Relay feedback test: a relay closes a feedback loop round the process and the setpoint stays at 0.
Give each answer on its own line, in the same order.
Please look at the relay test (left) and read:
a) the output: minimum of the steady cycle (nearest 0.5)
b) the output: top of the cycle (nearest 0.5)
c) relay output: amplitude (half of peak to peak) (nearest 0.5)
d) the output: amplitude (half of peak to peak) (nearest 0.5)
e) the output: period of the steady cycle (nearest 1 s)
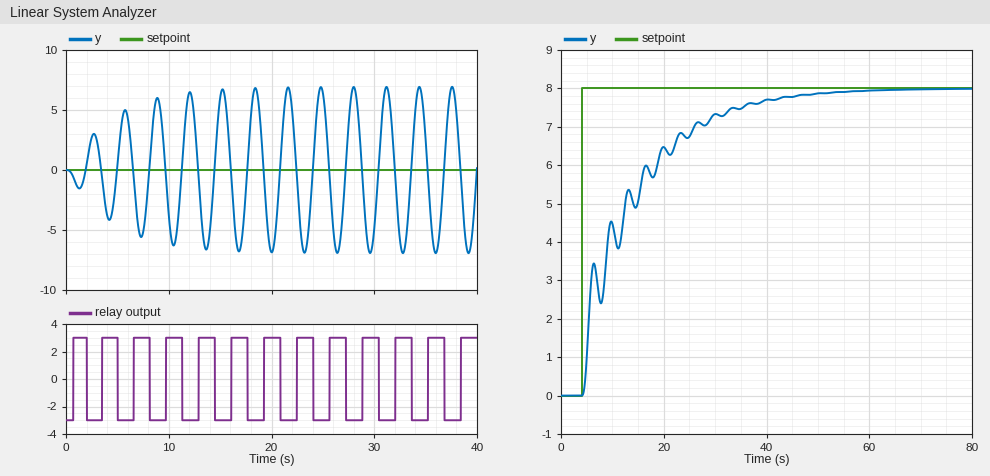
-7.0
7.0
3.0
7.0
3 s
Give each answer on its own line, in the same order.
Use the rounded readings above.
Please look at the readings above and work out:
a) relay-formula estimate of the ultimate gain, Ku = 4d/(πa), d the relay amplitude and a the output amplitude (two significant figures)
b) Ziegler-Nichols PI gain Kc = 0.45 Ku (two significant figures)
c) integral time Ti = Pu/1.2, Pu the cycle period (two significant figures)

0.55
0.25
2.5 s
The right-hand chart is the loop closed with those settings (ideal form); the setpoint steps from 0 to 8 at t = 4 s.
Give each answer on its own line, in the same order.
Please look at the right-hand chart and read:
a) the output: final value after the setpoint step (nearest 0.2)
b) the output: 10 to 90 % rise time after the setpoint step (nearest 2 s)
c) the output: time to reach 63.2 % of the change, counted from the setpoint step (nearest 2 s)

8.0
24 s
8 s
